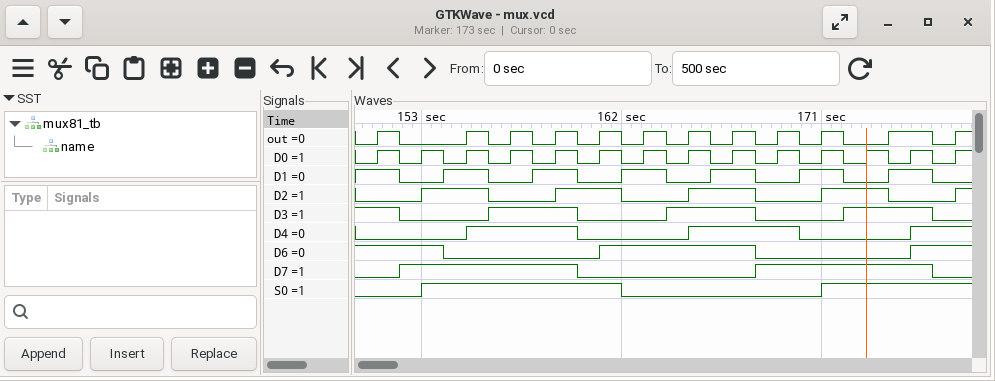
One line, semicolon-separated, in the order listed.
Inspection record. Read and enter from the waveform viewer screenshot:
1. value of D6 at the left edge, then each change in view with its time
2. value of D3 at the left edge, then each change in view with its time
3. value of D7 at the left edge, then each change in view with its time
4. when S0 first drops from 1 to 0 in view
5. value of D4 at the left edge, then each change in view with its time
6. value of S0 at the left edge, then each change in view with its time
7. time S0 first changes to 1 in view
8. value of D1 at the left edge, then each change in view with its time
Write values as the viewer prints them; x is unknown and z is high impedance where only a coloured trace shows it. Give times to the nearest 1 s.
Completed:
1, 0 at 154 s, 1 at 161 s, 0 at 168 s, 1 at 175 s; 1, 0 at 152 s, 1 at 156 s, 0 at 160 s, 1 at 164 s, 0 at 168 s, 1 at 172 s, 0 at 176 s; 0, 1 at 152 s, 0 at 160 s, 1 at 168 s, 0 at 176 s; 162 s; 0, 1 at 155 s, 0 at 160 s, 1 at 165 s, 0 at 170 s, 1 at 175 s; 0, 1 at 153 s, 0 at 162 s, 1 at 171 s; 153 s; 1, 0 at 152 s, 1 at 154 s, 0 at 156 s, 1 at 158 s, 0 at 160 s, 1 at 162 s, 0 at 164 s, 1 at 166 s, 0 at 168 s, 1 at 170 s, 0 at 172 s, 1 at 174 s, 0 at 176 s
